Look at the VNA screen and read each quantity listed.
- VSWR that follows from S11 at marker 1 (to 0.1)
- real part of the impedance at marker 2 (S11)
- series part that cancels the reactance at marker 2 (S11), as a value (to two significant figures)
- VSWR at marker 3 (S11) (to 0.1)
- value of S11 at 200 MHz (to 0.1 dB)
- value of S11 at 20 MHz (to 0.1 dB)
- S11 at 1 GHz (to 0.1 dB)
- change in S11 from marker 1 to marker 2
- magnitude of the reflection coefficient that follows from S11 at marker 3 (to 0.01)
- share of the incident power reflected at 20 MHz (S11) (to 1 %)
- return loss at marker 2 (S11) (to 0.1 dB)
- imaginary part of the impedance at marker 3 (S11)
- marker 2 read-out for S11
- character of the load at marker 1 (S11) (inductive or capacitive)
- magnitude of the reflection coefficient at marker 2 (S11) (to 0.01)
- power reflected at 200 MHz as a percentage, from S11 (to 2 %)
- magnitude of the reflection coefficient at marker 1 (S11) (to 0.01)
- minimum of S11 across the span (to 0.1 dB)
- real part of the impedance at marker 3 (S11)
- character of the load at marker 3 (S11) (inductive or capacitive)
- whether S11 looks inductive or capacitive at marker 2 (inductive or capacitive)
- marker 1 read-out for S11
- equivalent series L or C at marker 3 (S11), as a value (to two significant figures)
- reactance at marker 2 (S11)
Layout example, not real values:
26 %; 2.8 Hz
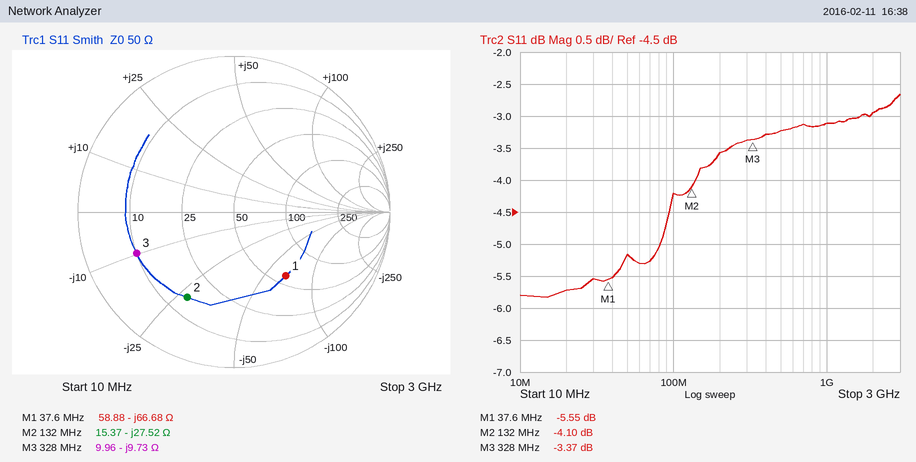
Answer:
3.2; 15.37 Ω; 33 nH; 5.2; -3.6 dB; -5.7 dB; -3.1 dB; 1.45 dB; 0.68; 27 %; 4.1 dB; -9.73 Ω; -4.10 dB; capacitive; 0.62; 44 %; 0.53; -5.8 dB; 9.96 Ω; capacitive; capacitive; -5.55 dB; 50 pF; -27.52 Ω
